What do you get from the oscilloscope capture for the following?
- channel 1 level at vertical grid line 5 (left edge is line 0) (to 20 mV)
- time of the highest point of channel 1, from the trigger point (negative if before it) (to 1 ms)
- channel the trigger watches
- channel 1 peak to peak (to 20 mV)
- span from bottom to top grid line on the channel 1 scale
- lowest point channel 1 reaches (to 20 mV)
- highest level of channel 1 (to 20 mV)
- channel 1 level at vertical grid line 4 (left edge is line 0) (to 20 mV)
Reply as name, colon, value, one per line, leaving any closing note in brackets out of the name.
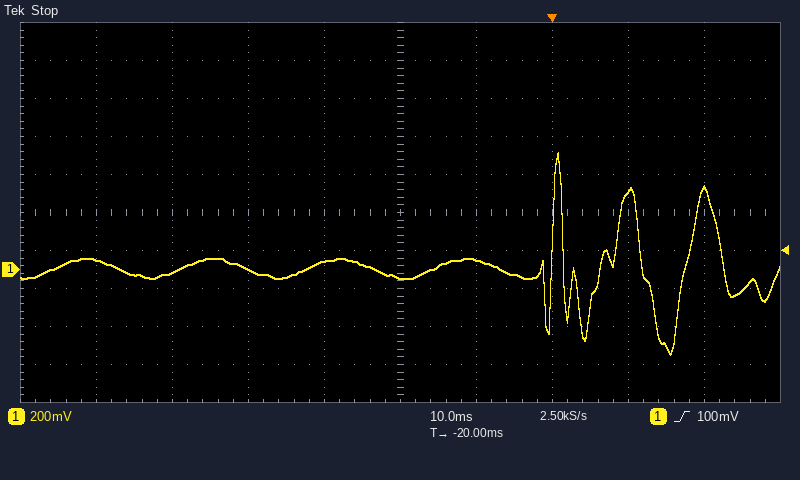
channel 1 level at vertical grid line 5 (left edge is line 0): -40 mV
time of the highest point of channel 1, from the trigger point (negative if before it): +1 ms
channel the trigger watches: channel 1
channel 1 peak to peak: 1.06 V
span from bottom to top grid line on the channel 1 scale: 2 V
lowest point channel 1 reaches: -440 mV
highest level of channel 1: 620 mV
channel 1 level at vertical grid line 4 (left edge is line 0): 40 mV
